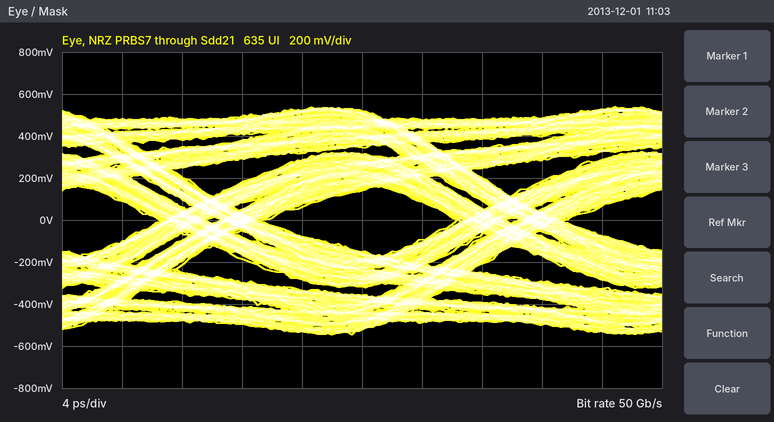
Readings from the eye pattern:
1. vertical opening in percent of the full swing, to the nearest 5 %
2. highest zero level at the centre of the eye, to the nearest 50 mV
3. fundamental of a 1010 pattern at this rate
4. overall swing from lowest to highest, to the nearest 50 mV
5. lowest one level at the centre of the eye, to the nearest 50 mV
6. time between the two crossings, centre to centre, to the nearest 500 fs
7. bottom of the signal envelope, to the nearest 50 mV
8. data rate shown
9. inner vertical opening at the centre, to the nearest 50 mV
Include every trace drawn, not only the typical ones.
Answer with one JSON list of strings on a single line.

["25 %", "-150 mV", "25 GHz", "1.10 V", "150 mV", "20.0 ps", "-550 mV", "50 Gb/s", "300 mV"]
